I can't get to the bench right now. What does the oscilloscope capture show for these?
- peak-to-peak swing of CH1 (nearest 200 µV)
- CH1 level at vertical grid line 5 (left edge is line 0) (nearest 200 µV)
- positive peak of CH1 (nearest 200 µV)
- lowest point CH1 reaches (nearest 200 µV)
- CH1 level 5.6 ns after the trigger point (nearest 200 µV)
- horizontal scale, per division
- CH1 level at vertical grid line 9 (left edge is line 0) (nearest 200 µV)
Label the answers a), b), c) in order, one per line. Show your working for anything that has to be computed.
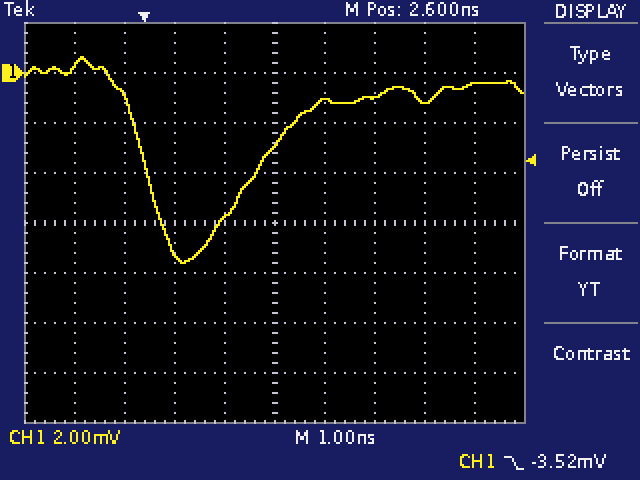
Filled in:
a) 600 µV − (-7.6 mV) = 8.2 mV
b) -3.0 mV
c) 600 µV
d) -7.6 mV
e) -1.2 mV
f) 1 ns
g) -400 µV
